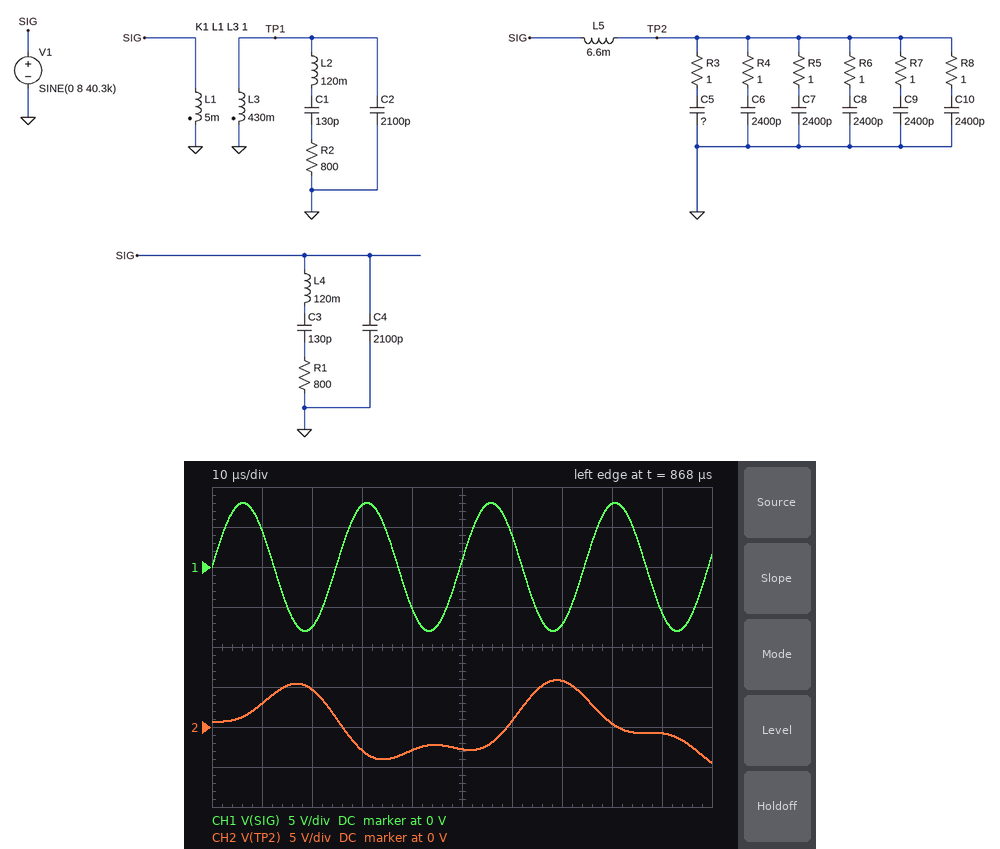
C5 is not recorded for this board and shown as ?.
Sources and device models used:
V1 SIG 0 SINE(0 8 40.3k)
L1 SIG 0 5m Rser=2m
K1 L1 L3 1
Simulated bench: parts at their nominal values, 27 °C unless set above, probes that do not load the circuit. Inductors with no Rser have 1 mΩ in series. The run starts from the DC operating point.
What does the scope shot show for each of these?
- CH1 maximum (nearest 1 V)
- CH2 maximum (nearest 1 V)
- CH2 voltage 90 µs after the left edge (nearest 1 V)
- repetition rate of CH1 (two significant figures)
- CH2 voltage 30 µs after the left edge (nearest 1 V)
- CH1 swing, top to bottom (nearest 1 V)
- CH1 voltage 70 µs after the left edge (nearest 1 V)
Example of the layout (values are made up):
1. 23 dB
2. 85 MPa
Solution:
1. 8 V
2. 6 V
3. -1 V
4. 40 kHz
5. -3 V
6. 16 V
7. -7 V
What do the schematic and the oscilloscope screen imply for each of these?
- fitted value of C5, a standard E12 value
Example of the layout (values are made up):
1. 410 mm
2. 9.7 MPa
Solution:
1. 820 pF
